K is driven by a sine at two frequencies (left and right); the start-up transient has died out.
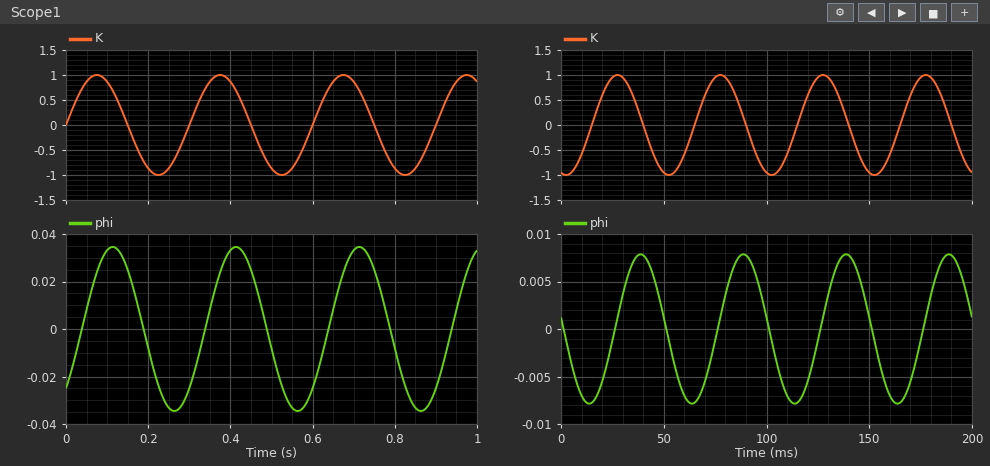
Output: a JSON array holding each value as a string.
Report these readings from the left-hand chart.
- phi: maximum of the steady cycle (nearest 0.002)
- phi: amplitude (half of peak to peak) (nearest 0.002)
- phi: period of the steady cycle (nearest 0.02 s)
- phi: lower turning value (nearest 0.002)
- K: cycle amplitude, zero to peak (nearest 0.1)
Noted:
["0.034", "0.034", "0.30 s", "-0.034", "1.0"]
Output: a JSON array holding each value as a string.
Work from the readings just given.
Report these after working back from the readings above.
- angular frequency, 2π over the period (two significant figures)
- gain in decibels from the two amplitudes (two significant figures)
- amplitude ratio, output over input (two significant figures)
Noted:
["21 rad/s", "-29 dB", "0.034"]
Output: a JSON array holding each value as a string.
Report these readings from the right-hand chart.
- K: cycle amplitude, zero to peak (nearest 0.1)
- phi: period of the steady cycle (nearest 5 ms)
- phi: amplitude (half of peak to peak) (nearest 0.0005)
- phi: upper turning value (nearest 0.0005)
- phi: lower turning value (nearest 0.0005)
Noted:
["1.0", "50 ms", "0.0080", "0.0080", "-0.0080"]
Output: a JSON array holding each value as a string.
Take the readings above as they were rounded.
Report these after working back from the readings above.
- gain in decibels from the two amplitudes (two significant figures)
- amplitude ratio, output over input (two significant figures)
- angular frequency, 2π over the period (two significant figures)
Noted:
["-42 dB", "0.0080", "0.13 rad/ms"]
